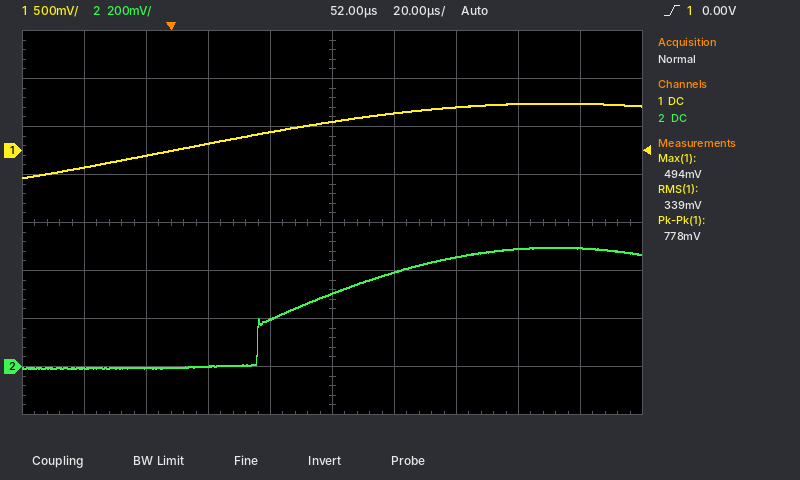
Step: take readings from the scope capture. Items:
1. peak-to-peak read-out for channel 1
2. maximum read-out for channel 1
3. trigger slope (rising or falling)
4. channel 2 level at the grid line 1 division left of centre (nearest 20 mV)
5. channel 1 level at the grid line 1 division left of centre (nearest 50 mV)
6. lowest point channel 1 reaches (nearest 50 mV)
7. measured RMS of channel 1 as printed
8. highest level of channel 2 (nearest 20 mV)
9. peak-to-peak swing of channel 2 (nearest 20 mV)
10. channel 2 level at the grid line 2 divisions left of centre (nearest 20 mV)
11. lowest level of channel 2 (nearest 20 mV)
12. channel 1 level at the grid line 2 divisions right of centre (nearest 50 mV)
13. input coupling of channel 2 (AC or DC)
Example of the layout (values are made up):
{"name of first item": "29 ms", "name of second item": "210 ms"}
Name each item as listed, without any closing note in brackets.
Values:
{"peak-to-peak read-out for channel 1": "778 mV", "maximum read-out for channel 1": "494 mV", "trigger slope": "rising", "channel 2 level at the grid line 1 division left of centre": "200 mV", "channel 1 level at the grid line 1 division left of centre": "200 mV", "lowest point channel 1 reaches": "-300 mV", "measured RMS of channel 1 as printed": "339 mV", "highest level of channel 2": "500 mV", "peak-to-peak swing of channel 2": "500 mV", "channel 2 level at the grid line 2 divisions left of centre": "0 mV", "lowest level of channel 2": "0 mV", "channel 1 level at the grid line 2 divisions right of centre": "450 mV", "input coupling of channel 2": "DC"}
